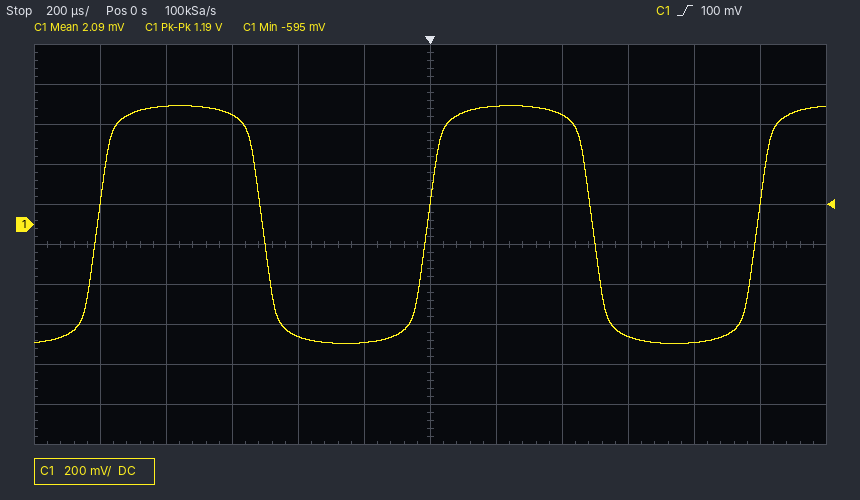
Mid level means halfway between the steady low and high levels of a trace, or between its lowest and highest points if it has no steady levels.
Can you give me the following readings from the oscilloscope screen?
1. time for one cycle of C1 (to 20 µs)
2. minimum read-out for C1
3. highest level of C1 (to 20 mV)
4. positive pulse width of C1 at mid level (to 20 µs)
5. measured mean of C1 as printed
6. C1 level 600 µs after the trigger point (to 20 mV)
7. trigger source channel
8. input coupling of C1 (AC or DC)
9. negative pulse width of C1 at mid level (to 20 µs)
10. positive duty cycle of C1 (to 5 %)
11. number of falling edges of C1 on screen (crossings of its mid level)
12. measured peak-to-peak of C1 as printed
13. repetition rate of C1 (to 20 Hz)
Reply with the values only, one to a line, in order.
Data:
1.00 ms
-595 mV
600 mV
500 µs
2.09 mV
-560 mV
C1
DC
500 µs
50 %
2
1.19 V
1.00 kHz
